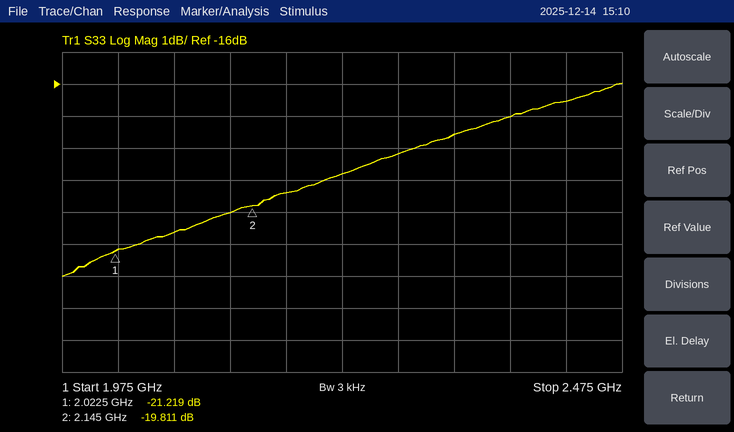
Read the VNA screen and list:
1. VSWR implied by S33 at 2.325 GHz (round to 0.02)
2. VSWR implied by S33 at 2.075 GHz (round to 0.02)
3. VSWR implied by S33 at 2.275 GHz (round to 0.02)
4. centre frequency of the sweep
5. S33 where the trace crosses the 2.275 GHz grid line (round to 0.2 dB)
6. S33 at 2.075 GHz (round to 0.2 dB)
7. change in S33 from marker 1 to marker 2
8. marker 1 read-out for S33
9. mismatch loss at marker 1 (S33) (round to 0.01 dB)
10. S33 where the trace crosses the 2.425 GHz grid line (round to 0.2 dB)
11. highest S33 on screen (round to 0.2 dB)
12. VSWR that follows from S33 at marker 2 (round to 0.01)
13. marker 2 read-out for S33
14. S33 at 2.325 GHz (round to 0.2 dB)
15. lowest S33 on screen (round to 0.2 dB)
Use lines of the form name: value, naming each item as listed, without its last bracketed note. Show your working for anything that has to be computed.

VSWR implied by S33 at 2.325 GHz: |Γ| = 10^(-17.6/20) = 0.1318; VSWR = (1 + 0.1318)/(1 − 0.1318) ≈ 1.30
VSWR implied by S33 at 2.075 GHz: |Γ| = 10^(-20.6/20) = 0.0933; VSWR = (1 + 0.0933)/(1 − 0.0933) ≈ 1.21, so 1.20 to the nearest 0.02
VSWR implied by S33 at 2.275 GHz: |Γ| = 10^(-18.2/20) = 0.1230; VSWR = (1 + 0.1230)/(1 − 0.1230) ≈ 1.28
centre frequency of the sweep: 2.225 GHz
S33 where the trace crosses the 2.275 GHz grid line: -18.2 dB
S33 at 2.075 GHz: -20.6 dB
change in S33 from marker 1 to marker 2: -19.811 − (-21.219) = 1.408 dB
marker 1 read-out for S33: -21.219 dB
mismatch loss at marker 1 (S33): −10 log10(1 − 10^(-21.219/10)) ≈ 0.03 dB
S33 where the trace crosses the 2.425 GHz grid line: -16.6 dB
highest S33 on screen: -16.0 dB
VSWR that follows from S33 at marker 2: (1 + 0.1022)/(1 − 0.1022) ≈ 1.23
marker 2 read-out for S33: -19.811 dB
S33 at 2.325 GHz: -17.6 dB
lowest S33 on screen: -22.0 dB
